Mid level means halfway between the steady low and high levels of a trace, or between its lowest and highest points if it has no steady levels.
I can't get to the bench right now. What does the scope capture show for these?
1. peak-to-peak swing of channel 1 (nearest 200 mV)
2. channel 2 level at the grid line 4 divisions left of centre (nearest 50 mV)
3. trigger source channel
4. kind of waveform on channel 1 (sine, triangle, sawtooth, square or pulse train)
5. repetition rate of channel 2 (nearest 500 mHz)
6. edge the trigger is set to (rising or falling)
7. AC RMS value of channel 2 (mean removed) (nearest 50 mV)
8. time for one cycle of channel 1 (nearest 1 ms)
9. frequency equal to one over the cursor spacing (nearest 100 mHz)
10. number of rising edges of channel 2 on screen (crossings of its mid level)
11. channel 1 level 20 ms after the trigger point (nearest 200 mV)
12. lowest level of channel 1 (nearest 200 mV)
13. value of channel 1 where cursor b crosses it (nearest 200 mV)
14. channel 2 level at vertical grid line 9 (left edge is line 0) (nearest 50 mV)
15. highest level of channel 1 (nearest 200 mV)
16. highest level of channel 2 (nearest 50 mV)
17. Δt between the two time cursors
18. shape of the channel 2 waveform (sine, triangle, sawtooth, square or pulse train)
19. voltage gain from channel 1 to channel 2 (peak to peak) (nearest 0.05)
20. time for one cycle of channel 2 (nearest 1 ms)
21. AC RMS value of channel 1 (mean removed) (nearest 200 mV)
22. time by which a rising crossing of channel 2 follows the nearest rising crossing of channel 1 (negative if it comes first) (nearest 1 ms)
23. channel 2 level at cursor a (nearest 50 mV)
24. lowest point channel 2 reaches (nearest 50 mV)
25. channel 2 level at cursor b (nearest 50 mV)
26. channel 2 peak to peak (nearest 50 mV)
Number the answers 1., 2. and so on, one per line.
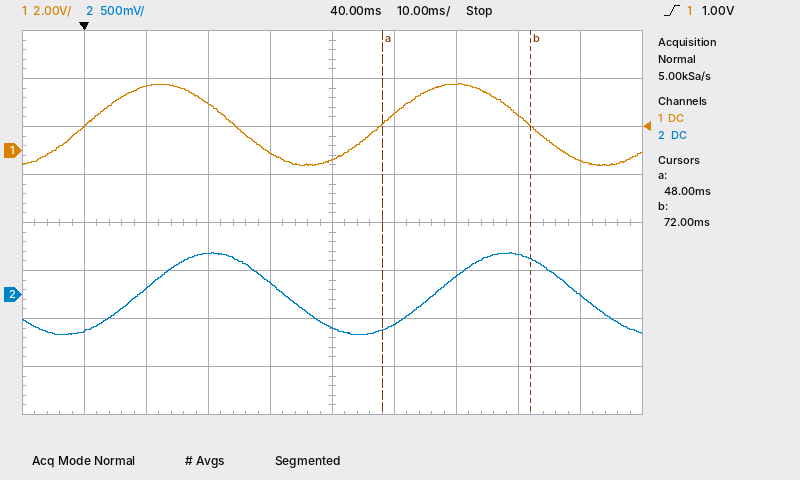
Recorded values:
1. 3.4 V
2. -400 mV
3. channel 1
4. sine
5. 21.0 Hz
6. rising
7. 300 mV
8. 48 ms
9. 41.7 Hz
10. 2
11. 2.0 V
12. -600 mV
13. 1.0 V
14. 0 mV
15. 2.8 V
16. 450 mV
17. 24 ms
18. sine
19. 0.25
20. 48 ms
21. 1.2 V
22. +9 ms
23. -350 mV
24. -400 mV
25. 350 mV
26. 850 mV
